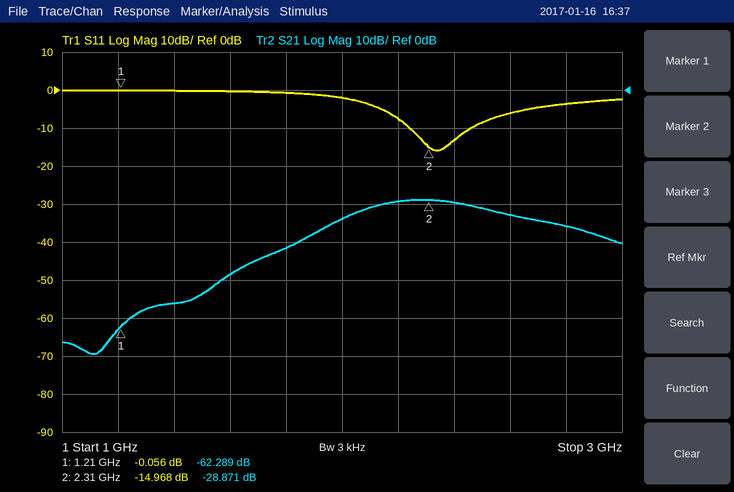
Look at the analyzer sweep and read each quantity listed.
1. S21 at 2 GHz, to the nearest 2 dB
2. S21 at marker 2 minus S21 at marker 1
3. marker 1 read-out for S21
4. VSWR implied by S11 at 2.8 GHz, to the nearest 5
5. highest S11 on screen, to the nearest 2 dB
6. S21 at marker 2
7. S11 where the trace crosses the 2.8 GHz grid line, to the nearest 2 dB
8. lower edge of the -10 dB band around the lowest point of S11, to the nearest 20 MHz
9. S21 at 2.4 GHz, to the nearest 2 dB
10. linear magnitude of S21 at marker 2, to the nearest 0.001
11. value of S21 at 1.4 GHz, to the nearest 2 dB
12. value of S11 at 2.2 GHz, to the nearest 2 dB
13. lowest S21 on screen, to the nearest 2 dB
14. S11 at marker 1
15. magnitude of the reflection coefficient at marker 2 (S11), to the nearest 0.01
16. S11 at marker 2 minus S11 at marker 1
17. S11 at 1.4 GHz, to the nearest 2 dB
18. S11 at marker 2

-34 dB
33.418 dB
-62.289 dB
5
0 dB
-28.871 dB
-4 dB
2.24 GHz
-30 dB
0.036
-56 dB
-8 dB
-70 dB
-0.056 dB
0.18
-14.912 dB
0 dB
-14.968 dB
